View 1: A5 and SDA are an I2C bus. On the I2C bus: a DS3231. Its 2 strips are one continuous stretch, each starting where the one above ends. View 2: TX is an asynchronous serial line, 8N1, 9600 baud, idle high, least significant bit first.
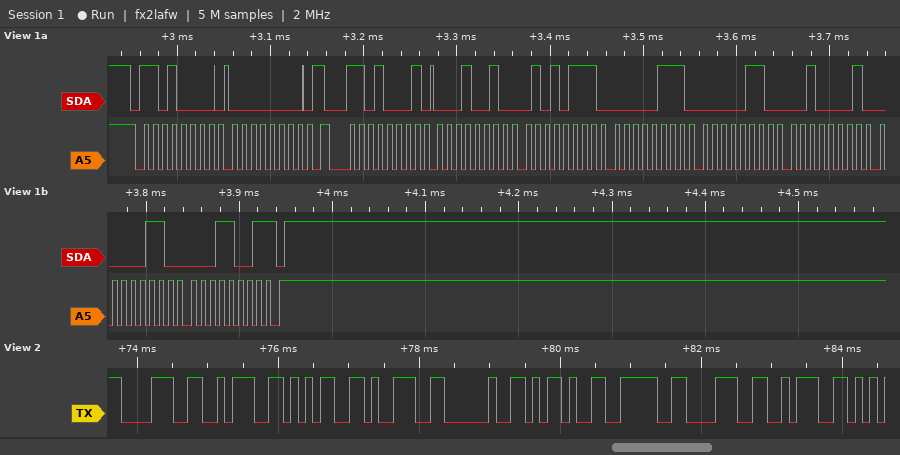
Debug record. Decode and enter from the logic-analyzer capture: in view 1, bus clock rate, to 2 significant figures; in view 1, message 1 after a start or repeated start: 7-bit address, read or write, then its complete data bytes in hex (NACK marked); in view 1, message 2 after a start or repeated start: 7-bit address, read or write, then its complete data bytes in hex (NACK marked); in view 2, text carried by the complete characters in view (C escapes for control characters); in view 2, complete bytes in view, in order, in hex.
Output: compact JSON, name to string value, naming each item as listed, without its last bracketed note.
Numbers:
{"in view 1, bus clock rate, to 2 significant figures": "100 kHz", "in view 1, message 1 after a start or repeated start: 7-bit address, read or write, then its complete data bytes in hex": "0x68 write: 00", "in view 1, message 2 after a start or repeated start: 7-bit address, read or write, then its complete data bytes in hex": "0x68 read: 12 57 07 06 21 06 19 NACK", "in view 2, text carried by the complete characters in view": "\"8:59 ->8:\"", "in view 2, complete bytes in view, in order, in hex": "38 3A 35 39 20 2D 3E 38 3A"}
